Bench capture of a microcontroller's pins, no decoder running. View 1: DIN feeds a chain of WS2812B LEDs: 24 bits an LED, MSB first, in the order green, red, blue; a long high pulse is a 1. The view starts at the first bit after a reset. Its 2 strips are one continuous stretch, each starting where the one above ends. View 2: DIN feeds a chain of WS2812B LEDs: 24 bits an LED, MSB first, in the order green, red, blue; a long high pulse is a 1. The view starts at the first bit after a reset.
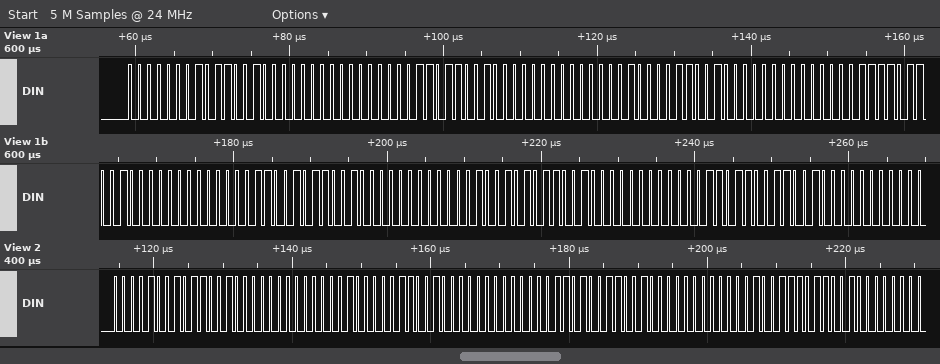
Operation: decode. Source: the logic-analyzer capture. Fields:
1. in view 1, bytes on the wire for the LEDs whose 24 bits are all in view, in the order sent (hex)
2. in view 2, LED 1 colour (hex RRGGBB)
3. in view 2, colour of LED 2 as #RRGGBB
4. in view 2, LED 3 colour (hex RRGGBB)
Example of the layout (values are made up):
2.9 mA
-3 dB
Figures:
01 64 00 03 64 00 08 64 00 0F 64 00 19 64 00 25 64 00 36 64 00
#640900
#641000
#641A00
